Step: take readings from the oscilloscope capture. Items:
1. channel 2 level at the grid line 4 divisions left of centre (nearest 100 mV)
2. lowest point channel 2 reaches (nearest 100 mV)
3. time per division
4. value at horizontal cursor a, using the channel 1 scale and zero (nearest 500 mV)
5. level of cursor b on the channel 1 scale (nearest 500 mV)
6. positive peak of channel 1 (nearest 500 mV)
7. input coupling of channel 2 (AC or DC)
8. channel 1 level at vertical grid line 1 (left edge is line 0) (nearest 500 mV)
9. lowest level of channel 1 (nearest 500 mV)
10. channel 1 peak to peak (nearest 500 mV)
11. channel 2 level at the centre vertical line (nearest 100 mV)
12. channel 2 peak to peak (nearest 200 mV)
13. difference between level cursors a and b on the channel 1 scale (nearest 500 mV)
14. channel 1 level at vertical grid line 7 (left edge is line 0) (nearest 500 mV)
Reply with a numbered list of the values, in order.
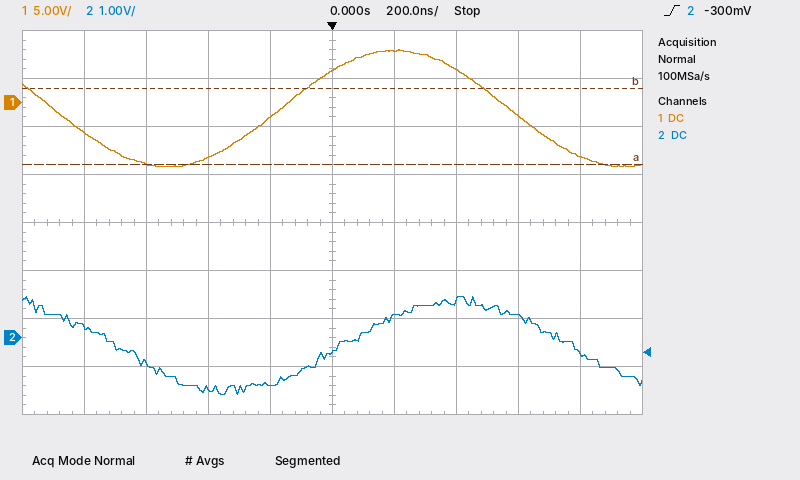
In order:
1. 200 mV
2. -1.2 V
3. 200 ns
4. -6.5 V
5. 1.5 V
6. 5.5 V
7. DC
8. -3.0 V
9. -6.5 V
10. 12.0 V
11. -300 mV
12. 2.0 V
13. 8.0 V
14. 3.5 V
